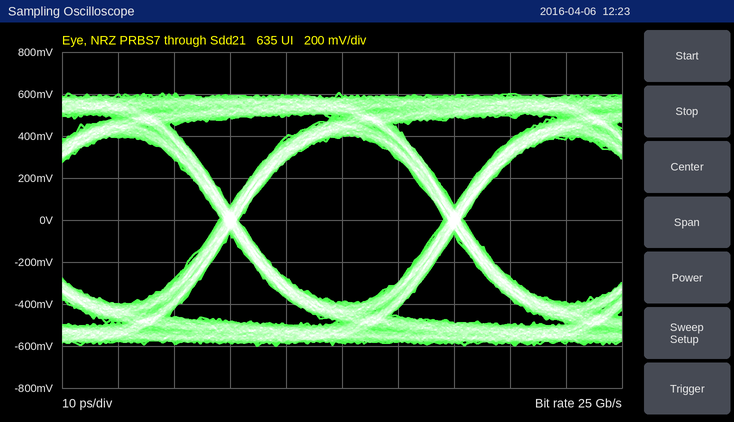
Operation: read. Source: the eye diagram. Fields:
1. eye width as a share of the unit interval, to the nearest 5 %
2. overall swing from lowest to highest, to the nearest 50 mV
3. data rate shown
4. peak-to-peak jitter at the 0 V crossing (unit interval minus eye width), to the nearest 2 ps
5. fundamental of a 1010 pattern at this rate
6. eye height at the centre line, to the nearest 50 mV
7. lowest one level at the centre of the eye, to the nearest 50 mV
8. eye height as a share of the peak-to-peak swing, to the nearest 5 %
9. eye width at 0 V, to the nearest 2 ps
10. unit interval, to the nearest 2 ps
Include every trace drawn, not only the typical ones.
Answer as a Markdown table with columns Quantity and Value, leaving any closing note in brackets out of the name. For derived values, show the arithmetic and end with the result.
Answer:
| Quantity | Value |
|---|---|
| eye width as a share of the unit interval, to the nearest 5 % | 36 ps / 40 ps ≈ 90 % |
| overall swing from lowest to highest, to the nearest 50 mV | 1.20 V |
| data rate shown | 25 Gb/s |
| peak-to-peak jitter at the 0 V crossing (unit interval minus eye width), to the nearest 2 ps | 4 ps |
| fundamental of a 1010 pattern at this rate | 12.5 GHz |
| eye height at the centre line, to the nearest 50 mV | 800 mV |
| lowest one level at the centre of the eye, to the nearest 50 mV | 400 mV |
| eye height as a share of the peak-to-peak swing, to the nearest 5 % | 800 mV / 1.20 V ≈ 66.7 %, so 65 % to the nearest 5 % |
| eye width at 0 V, to the nearest 2 ps | 36 ps |
| unit interval, to the nearest 2 ps | 40 ps |
